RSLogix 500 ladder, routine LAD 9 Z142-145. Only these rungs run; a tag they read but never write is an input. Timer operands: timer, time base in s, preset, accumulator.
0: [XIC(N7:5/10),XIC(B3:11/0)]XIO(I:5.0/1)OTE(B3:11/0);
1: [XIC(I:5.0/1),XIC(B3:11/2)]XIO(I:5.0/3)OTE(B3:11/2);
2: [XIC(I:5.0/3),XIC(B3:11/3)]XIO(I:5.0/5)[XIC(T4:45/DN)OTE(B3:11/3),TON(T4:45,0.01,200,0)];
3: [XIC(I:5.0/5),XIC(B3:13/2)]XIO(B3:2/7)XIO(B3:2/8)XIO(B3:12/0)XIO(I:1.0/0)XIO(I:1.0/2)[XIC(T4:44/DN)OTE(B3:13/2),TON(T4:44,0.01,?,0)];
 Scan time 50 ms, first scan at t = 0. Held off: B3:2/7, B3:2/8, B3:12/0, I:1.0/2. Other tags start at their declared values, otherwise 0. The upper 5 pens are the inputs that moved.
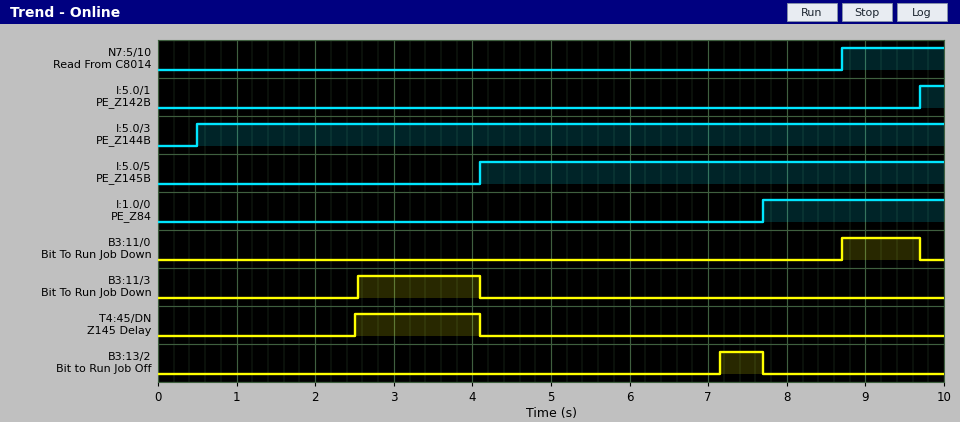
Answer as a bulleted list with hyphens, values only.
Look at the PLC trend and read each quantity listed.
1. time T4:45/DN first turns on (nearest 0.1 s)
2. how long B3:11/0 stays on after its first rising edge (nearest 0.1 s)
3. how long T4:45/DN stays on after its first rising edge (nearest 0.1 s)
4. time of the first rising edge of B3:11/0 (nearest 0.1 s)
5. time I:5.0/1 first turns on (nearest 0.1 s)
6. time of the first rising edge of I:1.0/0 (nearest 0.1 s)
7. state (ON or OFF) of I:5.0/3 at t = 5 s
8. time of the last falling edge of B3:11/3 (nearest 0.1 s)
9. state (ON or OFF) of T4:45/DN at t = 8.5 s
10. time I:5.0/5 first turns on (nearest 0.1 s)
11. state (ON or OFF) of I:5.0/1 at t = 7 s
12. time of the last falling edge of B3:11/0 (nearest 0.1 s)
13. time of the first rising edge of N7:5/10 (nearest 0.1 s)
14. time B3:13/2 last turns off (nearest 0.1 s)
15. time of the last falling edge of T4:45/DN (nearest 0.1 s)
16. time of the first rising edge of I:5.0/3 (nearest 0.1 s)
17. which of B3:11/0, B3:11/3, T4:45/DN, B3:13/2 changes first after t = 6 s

- 2.5 s
- 1.0 s
- 1.6 s
- 8.7 s
- 9.7 s
- 7.7 s
- ON
- 4.1 s
- OFF
- 4.1 s
- OFF
- 9.7 s
- 8.7 s
- 7.7 s
- 4.1 s
- 0.5 s
- B3:13/2
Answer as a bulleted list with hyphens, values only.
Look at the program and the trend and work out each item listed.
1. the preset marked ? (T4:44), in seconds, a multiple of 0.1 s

- 3.0 s
